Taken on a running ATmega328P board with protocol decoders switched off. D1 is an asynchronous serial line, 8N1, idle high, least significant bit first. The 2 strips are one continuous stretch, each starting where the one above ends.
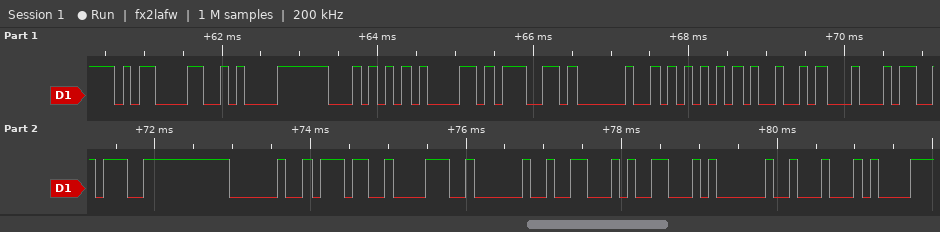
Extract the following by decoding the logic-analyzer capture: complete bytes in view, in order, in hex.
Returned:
0x0D 0x0A 0x54 0x61 0x67 0x20 0x55 0x49 0x44 0x3A 0x20 0x37 0x38 0x20 0x46 0x46 0x20 0x44
